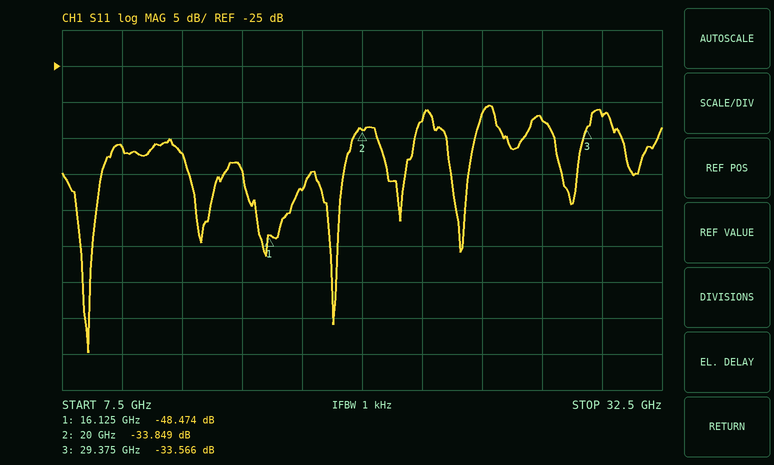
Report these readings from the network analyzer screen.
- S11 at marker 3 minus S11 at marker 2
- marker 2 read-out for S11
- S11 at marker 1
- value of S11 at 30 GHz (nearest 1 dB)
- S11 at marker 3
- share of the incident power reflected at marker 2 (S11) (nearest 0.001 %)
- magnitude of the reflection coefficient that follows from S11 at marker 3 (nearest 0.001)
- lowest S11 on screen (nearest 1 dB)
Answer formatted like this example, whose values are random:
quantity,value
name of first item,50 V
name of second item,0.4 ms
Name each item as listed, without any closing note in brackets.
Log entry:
quantity,value
S11 at marker 3 minus S11 at marker 2,0.283 dB
marker 2 read-out for S11,-33.849 dB
S11 at marker 1,-48.474 dB
value of S11 at 30 GHz,-32 dB
S11 at marker 3,-33.566 dB
share of the incident power reflected at marker 2 (S11),0.041 %
magnitude of the reflection coefficient that follows from S11 at marker 3,0.021
lowest S11 on screen,-65 dB
